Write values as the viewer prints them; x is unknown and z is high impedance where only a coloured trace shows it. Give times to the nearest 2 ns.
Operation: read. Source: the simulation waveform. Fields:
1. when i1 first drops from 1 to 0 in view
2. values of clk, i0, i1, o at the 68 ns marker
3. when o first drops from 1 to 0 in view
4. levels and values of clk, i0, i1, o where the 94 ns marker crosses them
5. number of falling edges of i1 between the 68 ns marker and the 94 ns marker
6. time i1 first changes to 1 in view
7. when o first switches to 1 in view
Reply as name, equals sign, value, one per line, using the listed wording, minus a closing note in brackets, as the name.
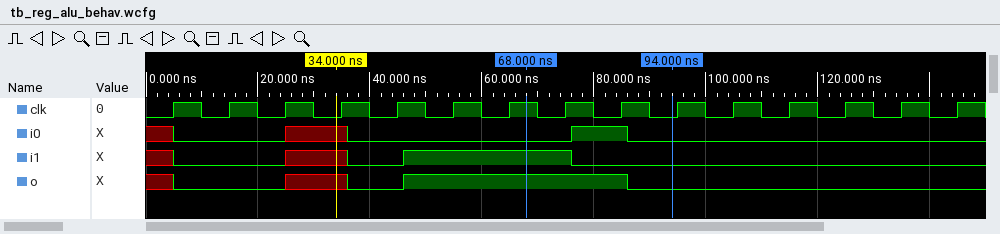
when i1 first drops from 1 to 0 in view = 76 ns
values of clk, i0, i1, o at the 68 ns marker = clk=1, i0=0, i1=1, o=1
when o first drops from 1 to 0 in view = 86 ns
levels and values of clk, i0, i1, o where the 94 ns marker crosses them = clk=0, i0=0, i1=0, o=0
number of falling edges of i1 between the 68 ns marker and the 94 ns marker = 1
time i1 first changes to 1 in view = 46 ns
when o first switches to 1 in view = 46 ns
